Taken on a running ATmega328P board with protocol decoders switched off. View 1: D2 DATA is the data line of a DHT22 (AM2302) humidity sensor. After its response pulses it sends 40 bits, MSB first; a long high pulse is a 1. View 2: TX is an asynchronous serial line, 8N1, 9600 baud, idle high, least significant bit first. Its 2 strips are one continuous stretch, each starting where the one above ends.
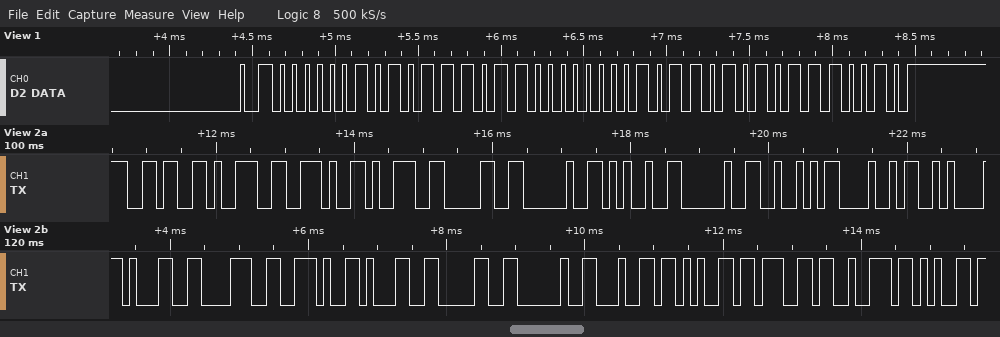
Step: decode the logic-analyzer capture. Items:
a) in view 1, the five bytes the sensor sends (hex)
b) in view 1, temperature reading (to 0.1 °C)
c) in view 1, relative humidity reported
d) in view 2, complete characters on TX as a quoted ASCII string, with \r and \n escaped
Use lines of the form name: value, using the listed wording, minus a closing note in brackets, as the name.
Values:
in view 1, the five bytes the sensor sends: 02 BB 00 B5 72
in view 1, temperature reading: 18.1 °C
in view 1, relative humidity reported: 69.9 %
in view 2, complete characters on TX as a quoted ASCII string, with \r and \n escaped: "69.90 % RH\n18.10 degre"
